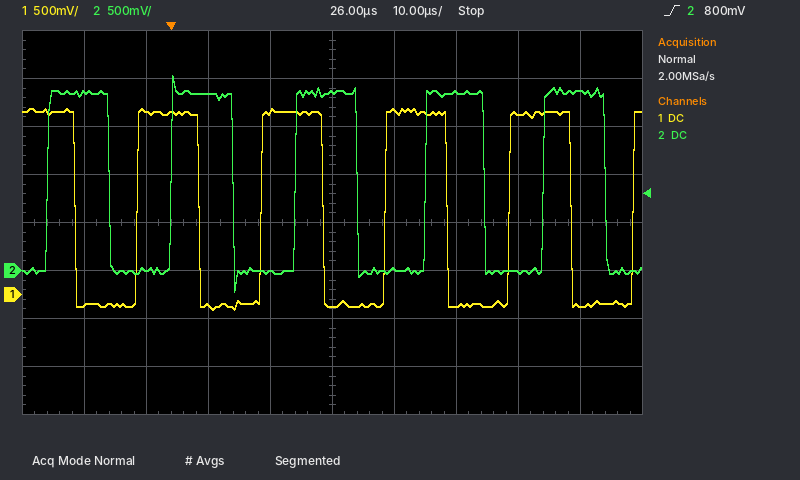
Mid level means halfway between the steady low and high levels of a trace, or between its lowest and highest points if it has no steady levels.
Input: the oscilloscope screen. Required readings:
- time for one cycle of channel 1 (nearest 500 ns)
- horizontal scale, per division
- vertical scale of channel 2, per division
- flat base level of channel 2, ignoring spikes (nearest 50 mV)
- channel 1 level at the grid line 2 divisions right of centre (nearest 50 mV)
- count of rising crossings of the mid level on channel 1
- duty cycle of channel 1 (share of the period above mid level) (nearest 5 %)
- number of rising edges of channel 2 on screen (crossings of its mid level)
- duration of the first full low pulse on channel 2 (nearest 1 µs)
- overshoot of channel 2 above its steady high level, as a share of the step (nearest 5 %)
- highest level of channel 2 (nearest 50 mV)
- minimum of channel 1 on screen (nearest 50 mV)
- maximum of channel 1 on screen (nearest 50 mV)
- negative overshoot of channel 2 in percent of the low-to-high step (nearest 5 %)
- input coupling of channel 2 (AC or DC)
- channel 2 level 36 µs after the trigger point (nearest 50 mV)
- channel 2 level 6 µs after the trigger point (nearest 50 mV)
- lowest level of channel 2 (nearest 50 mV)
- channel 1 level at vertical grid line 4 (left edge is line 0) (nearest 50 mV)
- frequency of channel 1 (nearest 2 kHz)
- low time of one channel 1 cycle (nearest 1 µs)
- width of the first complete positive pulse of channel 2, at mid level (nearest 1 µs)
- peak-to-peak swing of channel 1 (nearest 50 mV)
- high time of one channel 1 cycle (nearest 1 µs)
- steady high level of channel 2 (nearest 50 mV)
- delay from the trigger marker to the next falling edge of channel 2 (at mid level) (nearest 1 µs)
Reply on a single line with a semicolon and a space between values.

20.0 µs; 10 µs; 500 mV; 0 mV; -100 mV; 5; 50 %; 5; 10 µs; 10 %; 2.05 V; -150 mV; 1.95 V; 10 %; DC; 0 mV; 1.85 V; -200 mV; 1.90 V; 50 kHz; 10 µs; 10 µs; 2.10 V; 10 µs; 1.85 V; 10 µs
